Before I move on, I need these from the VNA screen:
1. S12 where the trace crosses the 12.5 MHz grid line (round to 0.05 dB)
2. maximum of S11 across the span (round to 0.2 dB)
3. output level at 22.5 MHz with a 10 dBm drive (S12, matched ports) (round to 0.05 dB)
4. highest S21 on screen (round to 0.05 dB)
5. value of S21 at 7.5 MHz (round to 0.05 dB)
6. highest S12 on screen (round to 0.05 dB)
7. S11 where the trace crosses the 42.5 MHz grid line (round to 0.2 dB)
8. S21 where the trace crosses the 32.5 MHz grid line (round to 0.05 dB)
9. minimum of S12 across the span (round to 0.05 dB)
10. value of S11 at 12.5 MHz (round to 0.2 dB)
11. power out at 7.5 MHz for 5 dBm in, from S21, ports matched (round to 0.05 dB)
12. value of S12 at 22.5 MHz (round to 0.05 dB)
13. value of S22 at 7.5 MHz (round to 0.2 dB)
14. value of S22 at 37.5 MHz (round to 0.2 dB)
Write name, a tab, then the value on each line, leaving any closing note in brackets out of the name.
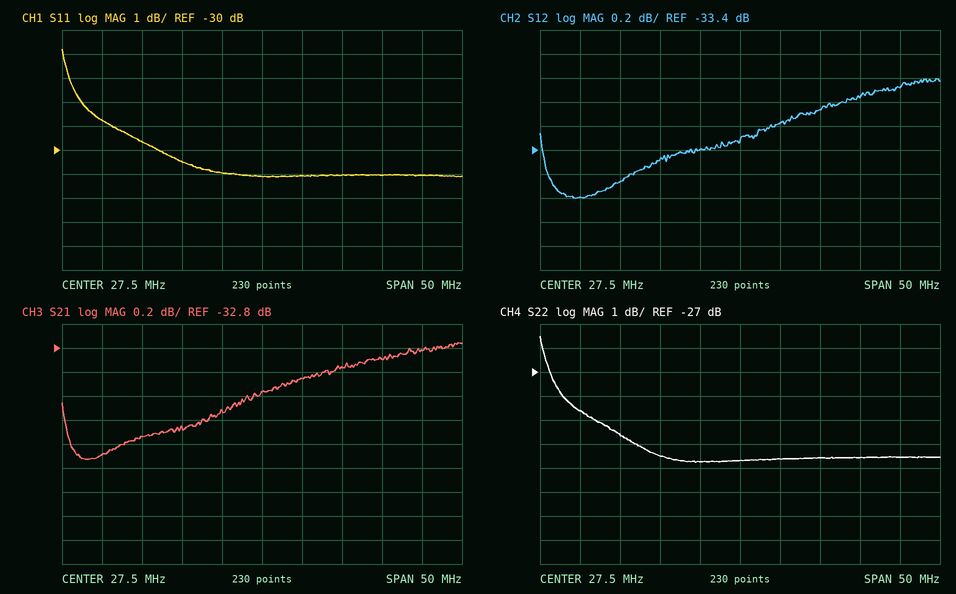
S12 where the trace crosses the 12.5 MHz grid line	-33.65 dB
maximum of S11 across the span	-25.8 dB
output level at 22.5 MHz with a 10 dBm drive (S12, matched ports)	-23.40 dBm
highest S21 on screen	-32.75 dB
value of S21 at 7.5 MHz	-33.70 dB
highest S12 on screen	-32.80 dB
S11 where the trace crosses the 42.5 MHz grid line	-31.0 dB
S21 where the trace crosses the 32.5 MHz grid line	-33.05 dB
minimum of S12 across the span	-33.80 dB
value of S11 at 12.5 MHz	-29.6 dB
power out at 7.5 MHz for 5 dBm in, from S21, ports matched	-28.70 dBm
value of S12 at 22.5 MHz	-33.40 dB
value of S22 at 7.5 MHz	-28.6 dB
value of S22 at 37.5 MHz	-30.6 dB
